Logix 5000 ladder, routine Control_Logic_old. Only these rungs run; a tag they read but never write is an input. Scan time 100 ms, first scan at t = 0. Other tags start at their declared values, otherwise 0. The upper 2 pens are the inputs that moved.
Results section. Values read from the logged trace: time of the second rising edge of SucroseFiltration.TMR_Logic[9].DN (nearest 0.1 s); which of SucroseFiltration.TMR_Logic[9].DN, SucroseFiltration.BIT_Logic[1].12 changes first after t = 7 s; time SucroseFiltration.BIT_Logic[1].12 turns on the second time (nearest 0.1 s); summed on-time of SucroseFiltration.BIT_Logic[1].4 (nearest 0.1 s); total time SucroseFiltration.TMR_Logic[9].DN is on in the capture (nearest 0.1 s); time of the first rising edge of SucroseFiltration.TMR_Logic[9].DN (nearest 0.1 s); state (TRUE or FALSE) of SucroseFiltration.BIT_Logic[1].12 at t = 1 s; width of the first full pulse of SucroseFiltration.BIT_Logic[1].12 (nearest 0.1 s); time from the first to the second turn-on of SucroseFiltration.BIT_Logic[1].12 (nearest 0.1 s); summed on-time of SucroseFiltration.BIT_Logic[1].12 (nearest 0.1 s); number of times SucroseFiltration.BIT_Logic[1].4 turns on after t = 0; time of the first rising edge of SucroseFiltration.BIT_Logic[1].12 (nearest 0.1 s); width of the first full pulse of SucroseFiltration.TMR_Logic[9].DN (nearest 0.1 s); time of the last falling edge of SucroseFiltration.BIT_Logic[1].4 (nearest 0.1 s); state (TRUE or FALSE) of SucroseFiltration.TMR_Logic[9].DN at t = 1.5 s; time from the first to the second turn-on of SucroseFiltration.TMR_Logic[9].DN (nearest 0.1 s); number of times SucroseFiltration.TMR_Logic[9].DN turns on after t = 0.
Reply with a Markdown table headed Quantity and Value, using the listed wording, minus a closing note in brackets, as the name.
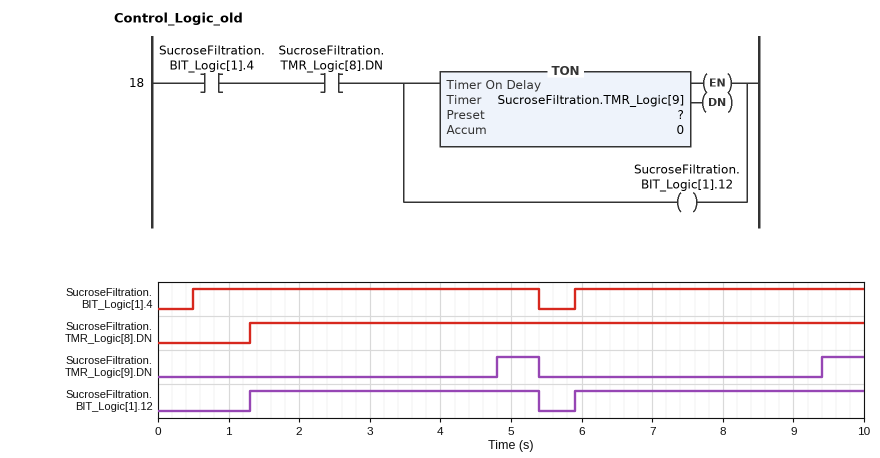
| Quantity | Value |
|---|---|
| time of the second rising edge of SucroseFiltration.TMR_Logic[9].DN | 9.4 s |
| which of SucroseFiltration.TMR_Logic[9].DN, SucroseFiltration.BIT_Logic[1].12 changes first after t = 7 s | SucroseFiltration.TMR_Logic[9].DN |
| time SucroseFiltration.BIT_Logic[1].12 turns on the second time | 5.9 s |
| summed on-time of SucroseFiltration.BIT_Logic[1].4 | 9.0 s |
| total time SucroseFiltration.TMR_Logic[9].DN is on in the capture | 1.2 s |
| time of the first rising edge of SucroseFiltration.TMR_Logic[9].DN | 4.8 s |
| state (TRUE or FALSE) of SucroseFiltration.BIT_Logic[1].12 at t = 1 s | FALSE |
| width of the first full pulse of SucroseFiltration.BIT_Logic[1].12 | 4.1 s |
| time from the first to the second turn-on of SucroseFiltration.BIT_Logic[1].12 | 4.6 s |
| summed on-time of SucroseFiltration.BIT_Logic[1].12 | 8.2 s |
| number of times SucroseFiltration.BIT_Logic[1].4 turns on after t = 0 | 2 |
| time of the first rising edge of SucroseFiltration.BIT_Logic[1].12 | 1.3 s |
| width of the first full pulse of SucroseFiltration.TMR_Logic[9].DN | 0.6 s |
| time of the last falling edge of SucroseFiltration.BIT_Logic[1].4 | 5.4 s |
| state (TRUE or FALSE) of SucroseFiltration.TMR_Logic[9].DN at t = 1.5 s | FALSE |
| time from the first to the second turn-on of SucroseFiltration.TMR_Logic[9].DN | 4.6 s |
| number of times SucroseFiltration.TMR_Logic[9].DN turns on after t = 0 | 2 |
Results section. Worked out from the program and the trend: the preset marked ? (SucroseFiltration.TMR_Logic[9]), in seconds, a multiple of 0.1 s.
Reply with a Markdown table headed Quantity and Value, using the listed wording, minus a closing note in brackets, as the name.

| Quantity | Value |
|---|---|
| the preset marked ? (SucroseFiltration.TMR_Logic[9]), in seconds, a multiple of 0.1 s | 3.5 s |
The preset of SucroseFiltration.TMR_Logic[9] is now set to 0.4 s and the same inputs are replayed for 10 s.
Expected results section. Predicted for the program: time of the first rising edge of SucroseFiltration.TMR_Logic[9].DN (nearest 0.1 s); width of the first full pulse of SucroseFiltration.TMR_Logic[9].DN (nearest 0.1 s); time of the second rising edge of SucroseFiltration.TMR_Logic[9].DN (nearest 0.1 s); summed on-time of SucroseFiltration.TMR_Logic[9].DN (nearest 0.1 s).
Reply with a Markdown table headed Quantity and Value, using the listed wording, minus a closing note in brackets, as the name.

| Quantity | Value |
|---|---|
| time of the first rising edge of SucroseFiltration.TMR_Logic[9].DN | 1.7 s |
| width of the first full pulse of SucroseFiltration.TMR_Logic[9].DN | 3.7 s |
| time of the second rising edge of SucroseFiltration.TMR_Logic[9].DN | 6.3 s |
| summed on-time of SucroseFiltration.TMR_Logic[9].DN | 7.4 s |
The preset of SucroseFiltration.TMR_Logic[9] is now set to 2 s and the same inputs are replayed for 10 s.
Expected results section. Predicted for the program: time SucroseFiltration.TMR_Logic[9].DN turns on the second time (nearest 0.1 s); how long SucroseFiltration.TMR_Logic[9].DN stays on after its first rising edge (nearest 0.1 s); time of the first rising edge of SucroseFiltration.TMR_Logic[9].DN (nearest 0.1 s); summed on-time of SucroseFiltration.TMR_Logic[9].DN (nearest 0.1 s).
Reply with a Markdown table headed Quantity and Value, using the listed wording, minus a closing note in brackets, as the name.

| Quantity | Value |
|---|---|
| time SucroseFiltration.TMR_Logic[9].DN turns on the second time | 7.9 s |
| how long SucroseFiltration.TMR_Logic[9].DN stays on after its first rising edge | 2.1 s |
| time of the first rising edge of SucroseFiltration.TMR_Logic[9].DN | 3.3 s |
| summed on-time of SucroseFiltration.TMR_Logic[9].DN | 4.2 s |
